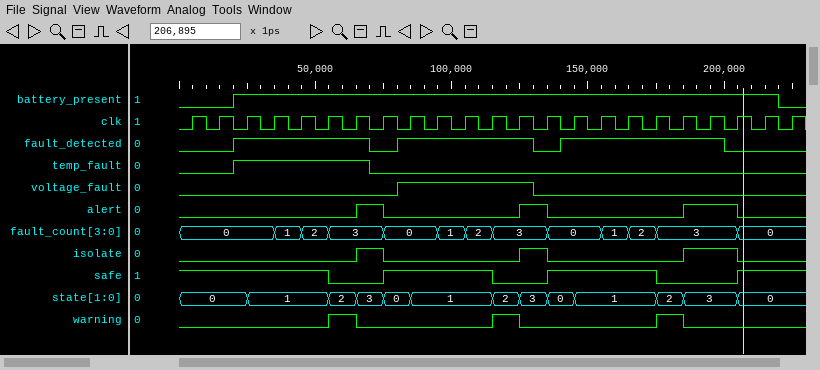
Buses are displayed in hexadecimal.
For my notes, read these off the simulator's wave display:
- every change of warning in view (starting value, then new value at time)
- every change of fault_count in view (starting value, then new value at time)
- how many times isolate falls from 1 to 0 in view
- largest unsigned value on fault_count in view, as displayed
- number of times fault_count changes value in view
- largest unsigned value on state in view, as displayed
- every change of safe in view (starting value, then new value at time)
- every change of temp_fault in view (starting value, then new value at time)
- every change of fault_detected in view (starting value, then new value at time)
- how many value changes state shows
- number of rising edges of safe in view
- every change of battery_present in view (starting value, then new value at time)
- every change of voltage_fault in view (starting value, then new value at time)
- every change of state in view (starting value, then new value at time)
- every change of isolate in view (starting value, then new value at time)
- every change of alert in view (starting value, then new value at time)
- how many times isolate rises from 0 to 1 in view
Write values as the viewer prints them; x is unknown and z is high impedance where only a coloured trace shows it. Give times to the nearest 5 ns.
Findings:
0, 1 at 55 ns, 0 at 65 ns, 1 at 115 ns, 0 at 125 ns, 1 at 175 ns, 0 at 185 ns
0, 1 at 35 ns, 2 at 45 ns, 3 at 55 ns, 0 at 75 ns, 1 at 95 ns, 2 at 105 ns, 3 at 115 ns, 0 at 135 ns, 1 at 155 ns, 2 at 165 ns, 3 at 175 ns, 0 at 205 ns
3
3
12
3
1, 0 at 55 ns, 1 at 75 ns, 0 at 115 ns, 1 at 135 ns, 0 at 175 ns, 1 at 205 ns
0, 1 at 20 ns, 0 at 70 ns
0, 1 at 20 ns, 0 at 70 ns, 1 at 80 ns, 0 at 130 ns, 1 at 140 ns, 0 at 200 ns
12
3
0, 1 at 20 ns, 0 at 220 ns
0, 1 at 80 ns, 0 at 130 ns
0, 1 at 25 ns, 2 at 55 ns, 3 at 65 ns, 0 at 75 ns, 1 at 85 ns, 2 at 115 ns, 3 at 125 ns, 0 at 135 ns, 1 at 145 ns, 2 at 175 ns, 3 at 185 ns, 0 at 205 ns
0, 1 at 65 ns, 0 at 75 ns, 1 at 125 ns, 0 at 135 ns, 1 at 185 ns, 0 at 205 ns
0, 1 at 65 ns, 0 at 75 ns, 1 at 125 ns, 0 at 135 ns, 1 at 185 ns, 0 at 205 ns
3
